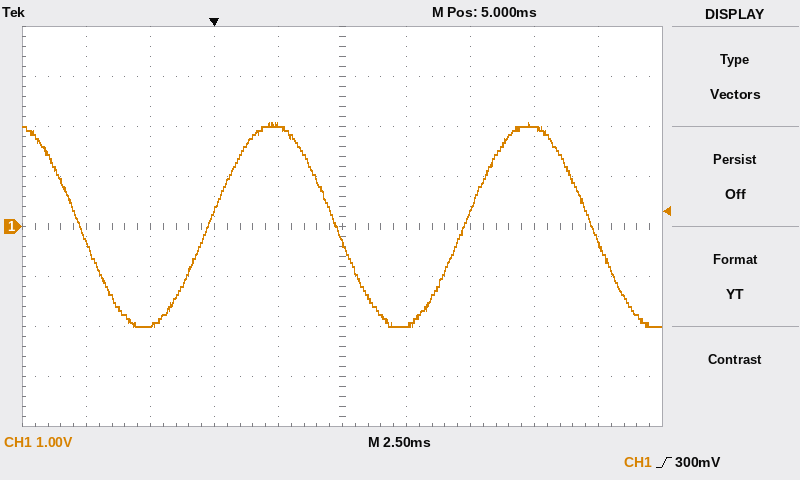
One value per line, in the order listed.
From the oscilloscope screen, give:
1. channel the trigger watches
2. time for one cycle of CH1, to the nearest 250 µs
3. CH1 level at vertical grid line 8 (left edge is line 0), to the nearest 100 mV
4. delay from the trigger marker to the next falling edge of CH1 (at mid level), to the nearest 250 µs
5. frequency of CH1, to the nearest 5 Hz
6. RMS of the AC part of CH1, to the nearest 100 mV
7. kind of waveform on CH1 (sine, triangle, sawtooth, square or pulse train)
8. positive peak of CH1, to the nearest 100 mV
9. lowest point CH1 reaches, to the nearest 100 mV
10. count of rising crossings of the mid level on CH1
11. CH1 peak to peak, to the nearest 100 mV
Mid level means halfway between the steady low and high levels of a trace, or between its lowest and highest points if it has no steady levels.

CH1
10.00 ms
2.0 V
4.75 ms
100 Hz
1.4 V
sine
2.1 V
-2.0 V
2
4.1 V
